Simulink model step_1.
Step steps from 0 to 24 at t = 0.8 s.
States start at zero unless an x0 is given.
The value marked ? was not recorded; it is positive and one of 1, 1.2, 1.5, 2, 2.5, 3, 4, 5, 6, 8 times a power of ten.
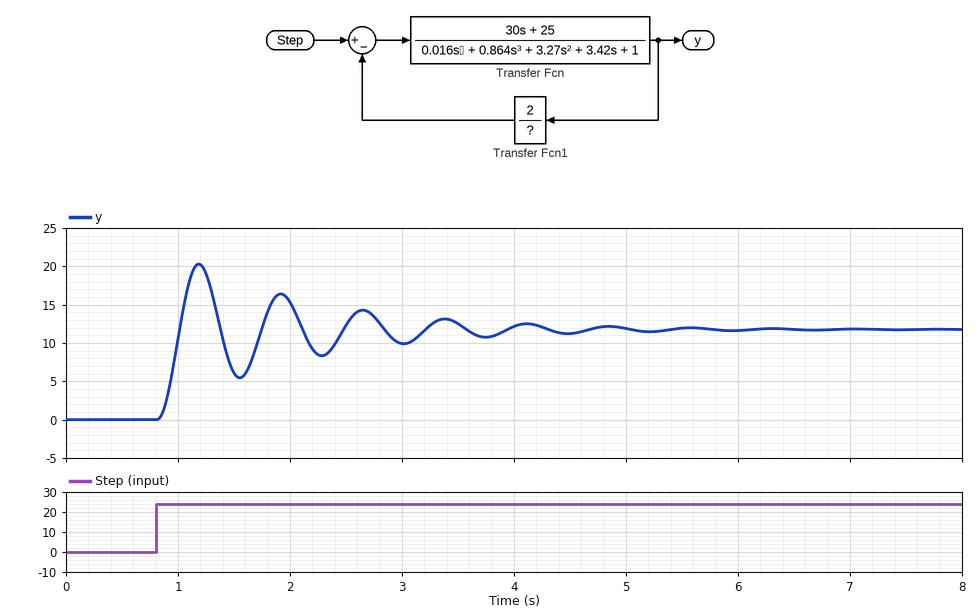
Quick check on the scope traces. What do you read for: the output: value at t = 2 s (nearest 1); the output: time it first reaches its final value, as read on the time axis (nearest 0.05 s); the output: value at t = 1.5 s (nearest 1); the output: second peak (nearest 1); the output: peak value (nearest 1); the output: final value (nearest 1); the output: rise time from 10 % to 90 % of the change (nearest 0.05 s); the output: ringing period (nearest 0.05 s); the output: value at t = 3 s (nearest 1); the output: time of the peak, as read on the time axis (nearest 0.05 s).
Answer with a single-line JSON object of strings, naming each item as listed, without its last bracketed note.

{"the output: value at t = 2 s": "15", "the output: time it first reaches its final value, as read on the time axis": "1.00 s", "the output: value at t = 1.5 s": "6", "the output: second peak": "16", "the output: peak value": "20", "the output: final value": "12", "the output: rise time from 10 % to 90 % of the change": "0.15 s", "the output: ringing period": "0.75 s", "the output: value at t = 3 s": "10", "the output: time of the peak, as read on the time axis": "1.20 s"}
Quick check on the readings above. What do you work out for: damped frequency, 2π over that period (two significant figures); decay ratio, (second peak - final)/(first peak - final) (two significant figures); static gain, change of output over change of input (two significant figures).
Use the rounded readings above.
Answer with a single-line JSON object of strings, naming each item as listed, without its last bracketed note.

{"damped frequency, 2π over that period": "8.4 rad/s", "decay ratio, (second peak - final)/(first peak - final)": "0.50", "static gain, change of output over change of input": "0.50"}
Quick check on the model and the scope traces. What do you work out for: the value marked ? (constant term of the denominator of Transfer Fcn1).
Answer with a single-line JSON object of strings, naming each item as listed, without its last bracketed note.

{"the value marked ?": "1"}
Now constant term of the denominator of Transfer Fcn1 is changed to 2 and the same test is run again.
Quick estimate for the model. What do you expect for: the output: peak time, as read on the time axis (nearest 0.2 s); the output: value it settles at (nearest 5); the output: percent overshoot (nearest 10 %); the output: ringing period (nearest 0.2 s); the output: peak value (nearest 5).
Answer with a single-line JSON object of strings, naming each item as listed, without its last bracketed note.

{"the output: peak time, as read on the time axis": "1.4 s", "the output: value it settles at": "25", "the output: percent overshoot": "50 %", "the output: ringing period": "1.0 s", "the output: peak value": "35"}
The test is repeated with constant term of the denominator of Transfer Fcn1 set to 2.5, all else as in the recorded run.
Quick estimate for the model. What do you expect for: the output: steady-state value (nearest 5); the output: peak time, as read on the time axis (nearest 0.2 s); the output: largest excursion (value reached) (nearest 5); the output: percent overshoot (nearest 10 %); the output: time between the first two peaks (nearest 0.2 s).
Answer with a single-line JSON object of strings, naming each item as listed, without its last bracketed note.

{"the output: steady-state value": "30", "the output: peak time, as read on the time axis": "1.4 s", "the output: largest excursion (value reached)": "40", "the output: percent overshoot": "50 %", "the output: time between the first two peaks": "1.2 s"}
